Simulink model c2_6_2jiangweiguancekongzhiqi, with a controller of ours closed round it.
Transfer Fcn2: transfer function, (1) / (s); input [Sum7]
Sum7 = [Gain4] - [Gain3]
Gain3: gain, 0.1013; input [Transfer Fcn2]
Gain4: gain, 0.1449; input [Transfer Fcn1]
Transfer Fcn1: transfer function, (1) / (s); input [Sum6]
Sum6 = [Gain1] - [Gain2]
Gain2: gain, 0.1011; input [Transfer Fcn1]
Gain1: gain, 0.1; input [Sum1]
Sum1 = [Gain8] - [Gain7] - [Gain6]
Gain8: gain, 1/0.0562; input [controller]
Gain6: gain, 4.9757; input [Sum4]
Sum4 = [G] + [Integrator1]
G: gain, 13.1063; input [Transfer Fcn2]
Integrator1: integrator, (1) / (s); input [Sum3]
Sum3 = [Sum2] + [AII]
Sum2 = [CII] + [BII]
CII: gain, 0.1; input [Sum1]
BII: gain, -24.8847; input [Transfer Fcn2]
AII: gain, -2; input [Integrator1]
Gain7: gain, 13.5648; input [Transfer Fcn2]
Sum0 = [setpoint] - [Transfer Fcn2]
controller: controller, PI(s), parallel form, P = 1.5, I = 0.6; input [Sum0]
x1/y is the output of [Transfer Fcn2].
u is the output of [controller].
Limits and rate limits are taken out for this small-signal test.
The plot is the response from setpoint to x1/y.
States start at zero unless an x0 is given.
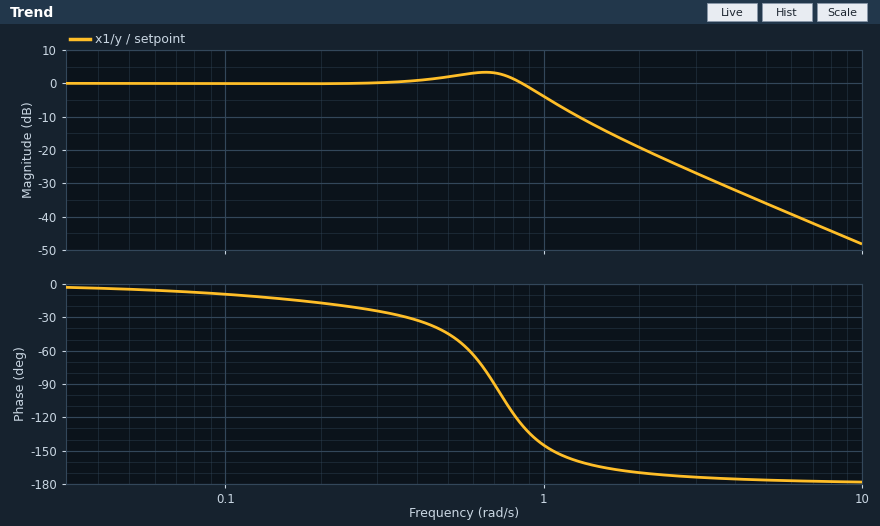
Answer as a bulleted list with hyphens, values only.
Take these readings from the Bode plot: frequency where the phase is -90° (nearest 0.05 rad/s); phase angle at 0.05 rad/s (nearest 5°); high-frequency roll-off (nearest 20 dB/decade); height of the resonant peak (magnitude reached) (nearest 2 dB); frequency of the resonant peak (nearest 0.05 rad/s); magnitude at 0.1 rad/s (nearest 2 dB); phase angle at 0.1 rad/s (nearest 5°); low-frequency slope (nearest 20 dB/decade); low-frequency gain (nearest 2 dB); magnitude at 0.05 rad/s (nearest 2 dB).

- 0.70 rad/s
- -5°
- -40 dB/decade
- 4 dB
- 0.65 rad/s
- 0 dB
- -10°
- 0 dB/decade
- 0 dB
- 0 dB
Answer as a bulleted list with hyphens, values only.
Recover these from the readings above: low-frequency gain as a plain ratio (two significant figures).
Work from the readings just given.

- 1.0
